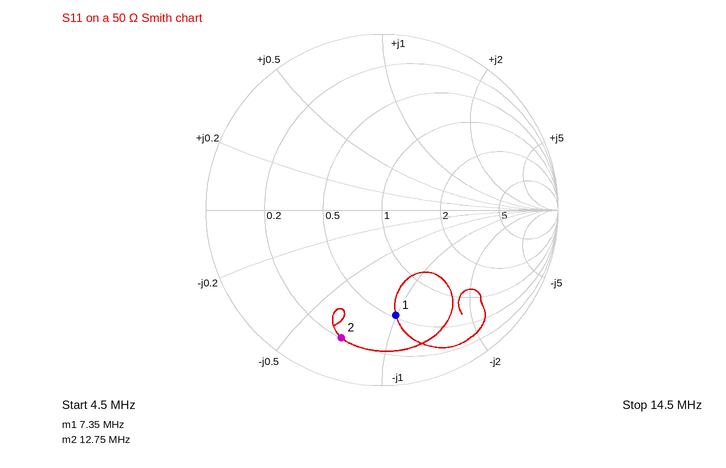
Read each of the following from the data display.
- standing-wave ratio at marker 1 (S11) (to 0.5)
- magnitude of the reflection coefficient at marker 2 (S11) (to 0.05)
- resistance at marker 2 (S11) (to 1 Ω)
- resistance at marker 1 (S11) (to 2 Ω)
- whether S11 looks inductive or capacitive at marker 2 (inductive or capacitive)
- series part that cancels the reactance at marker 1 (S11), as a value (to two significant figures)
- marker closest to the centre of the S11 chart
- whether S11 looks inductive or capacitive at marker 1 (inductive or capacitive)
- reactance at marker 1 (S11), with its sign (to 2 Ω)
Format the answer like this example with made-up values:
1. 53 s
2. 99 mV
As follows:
1. 4.0
2. 0.75
3. 10 Ω
4. 26 Ω
5. capacitive
6. 1.1 µH
7. marker 1
8. capacitive
9. -50 Ω
